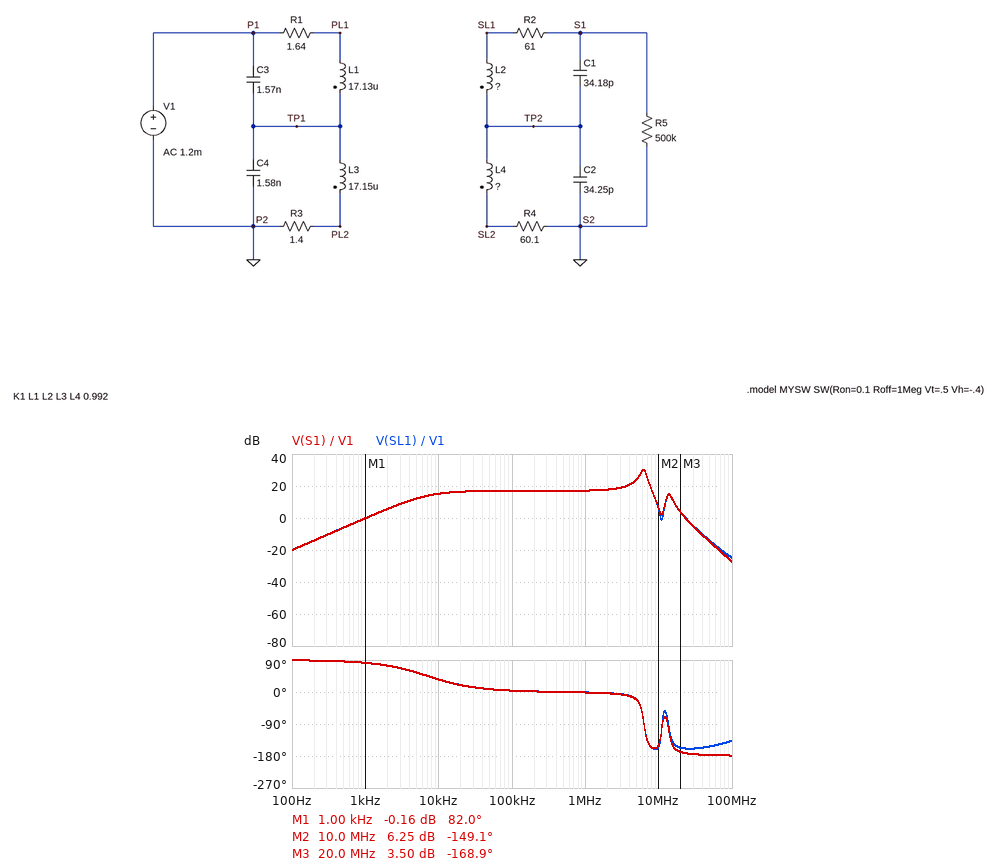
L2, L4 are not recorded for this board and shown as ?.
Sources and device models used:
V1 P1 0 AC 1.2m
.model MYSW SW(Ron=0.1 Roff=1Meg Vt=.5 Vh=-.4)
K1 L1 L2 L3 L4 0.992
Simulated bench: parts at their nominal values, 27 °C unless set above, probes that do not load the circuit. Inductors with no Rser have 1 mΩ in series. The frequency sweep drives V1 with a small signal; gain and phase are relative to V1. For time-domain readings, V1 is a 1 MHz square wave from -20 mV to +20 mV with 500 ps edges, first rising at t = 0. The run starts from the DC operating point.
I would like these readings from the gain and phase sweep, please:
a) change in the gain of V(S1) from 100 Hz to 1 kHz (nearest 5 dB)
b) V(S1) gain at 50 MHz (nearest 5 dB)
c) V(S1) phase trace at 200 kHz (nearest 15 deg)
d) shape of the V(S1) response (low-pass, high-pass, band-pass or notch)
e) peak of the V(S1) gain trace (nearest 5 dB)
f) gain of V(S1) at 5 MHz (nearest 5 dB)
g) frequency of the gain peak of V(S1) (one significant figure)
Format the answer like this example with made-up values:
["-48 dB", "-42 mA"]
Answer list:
["20 dB", "-15 dB", "0 deg", "band-pass", "30 dB", "25 dB", "6 MHz"]
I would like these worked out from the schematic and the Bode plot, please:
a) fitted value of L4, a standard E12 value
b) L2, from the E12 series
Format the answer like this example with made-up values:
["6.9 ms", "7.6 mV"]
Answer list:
["1.5 mH", "390 µH"]
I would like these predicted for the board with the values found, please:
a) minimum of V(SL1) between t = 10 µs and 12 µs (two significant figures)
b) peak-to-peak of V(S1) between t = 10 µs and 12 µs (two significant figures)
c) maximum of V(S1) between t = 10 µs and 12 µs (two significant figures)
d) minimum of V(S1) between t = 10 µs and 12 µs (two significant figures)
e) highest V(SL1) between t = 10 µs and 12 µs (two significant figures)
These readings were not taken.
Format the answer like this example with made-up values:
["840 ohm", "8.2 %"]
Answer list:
["-210 mV", "590 mV", "380 mV", "-210 mV", "380 mV"]
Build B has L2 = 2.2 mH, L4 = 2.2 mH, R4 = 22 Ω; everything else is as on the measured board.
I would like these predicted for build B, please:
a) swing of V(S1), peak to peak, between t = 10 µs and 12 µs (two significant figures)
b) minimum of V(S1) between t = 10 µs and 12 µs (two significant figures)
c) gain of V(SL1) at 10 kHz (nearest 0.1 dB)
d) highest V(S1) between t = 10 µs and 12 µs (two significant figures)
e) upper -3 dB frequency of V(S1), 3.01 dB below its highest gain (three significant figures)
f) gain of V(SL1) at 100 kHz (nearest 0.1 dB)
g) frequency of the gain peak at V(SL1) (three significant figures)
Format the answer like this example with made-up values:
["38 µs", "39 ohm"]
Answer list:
["1.1 V", "-400 mV", "19.3 dB", "680 mV", "5.05 MHz", "21.0 dB", "4.53 MHz"]
